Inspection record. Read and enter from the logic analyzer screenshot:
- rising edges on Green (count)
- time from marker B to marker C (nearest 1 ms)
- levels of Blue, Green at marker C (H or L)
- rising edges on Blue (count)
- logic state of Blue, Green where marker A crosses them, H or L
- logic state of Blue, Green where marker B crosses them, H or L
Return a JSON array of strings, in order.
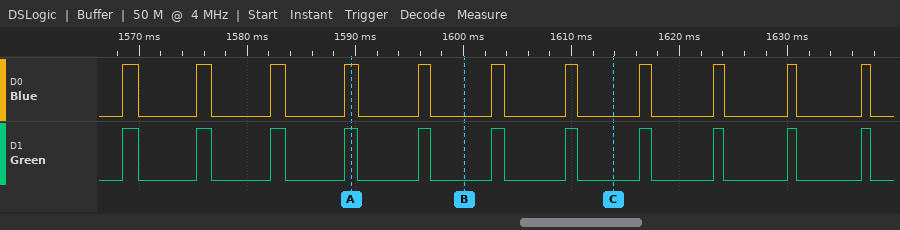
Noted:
["11", "14 ms", "Blue=L, Green=L", "11", "Blue=H, Green=H", "Blue=L, Green=L"]
